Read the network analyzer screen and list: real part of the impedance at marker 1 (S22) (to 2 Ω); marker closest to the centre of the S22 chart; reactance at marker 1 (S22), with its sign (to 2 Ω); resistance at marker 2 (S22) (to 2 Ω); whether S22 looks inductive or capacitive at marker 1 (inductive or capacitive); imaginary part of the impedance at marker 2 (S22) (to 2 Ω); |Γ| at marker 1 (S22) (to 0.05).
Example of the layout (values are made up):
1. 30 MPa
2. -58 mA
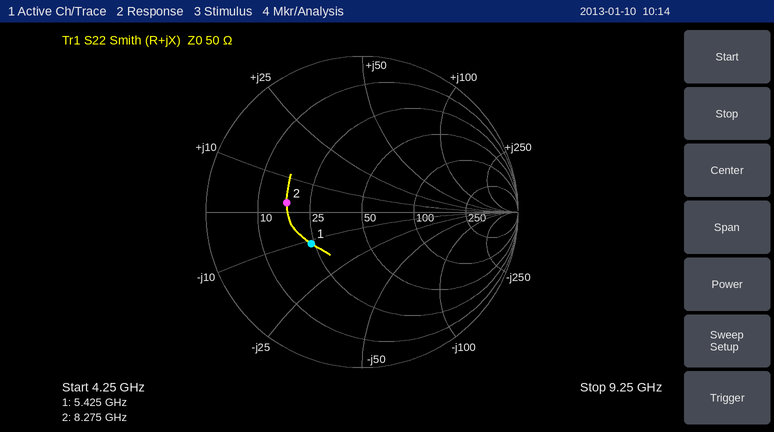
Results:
1. 24 Ω
2. marker 1
3. -12 Ω
4. 18 Ω
5. capacitive
6. +2 Ω
7. 0.40
